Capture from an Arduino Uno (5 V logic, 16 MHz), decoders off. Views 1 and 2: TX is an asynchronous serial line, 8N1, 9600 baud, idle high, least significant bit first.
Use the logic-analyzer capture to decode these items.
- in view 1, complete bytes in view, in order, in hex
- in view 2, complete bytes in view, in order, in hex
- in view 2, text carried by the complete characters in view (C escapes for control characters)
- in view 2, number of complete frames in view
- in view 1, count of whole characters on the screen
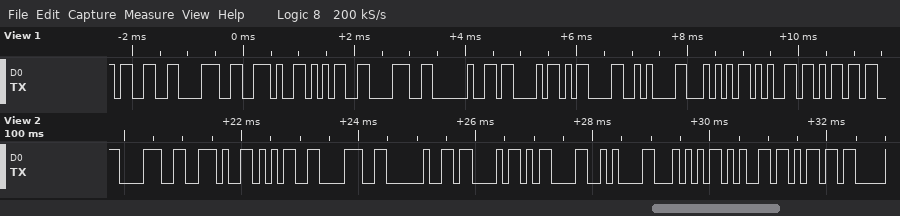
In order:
33 38 2E 35 38 20 43 0D 0A 54 65 6D
38 2E 35 38 20 43 0D 0A 54 65 6D
"8.58 C\r\nTem"
11
12
